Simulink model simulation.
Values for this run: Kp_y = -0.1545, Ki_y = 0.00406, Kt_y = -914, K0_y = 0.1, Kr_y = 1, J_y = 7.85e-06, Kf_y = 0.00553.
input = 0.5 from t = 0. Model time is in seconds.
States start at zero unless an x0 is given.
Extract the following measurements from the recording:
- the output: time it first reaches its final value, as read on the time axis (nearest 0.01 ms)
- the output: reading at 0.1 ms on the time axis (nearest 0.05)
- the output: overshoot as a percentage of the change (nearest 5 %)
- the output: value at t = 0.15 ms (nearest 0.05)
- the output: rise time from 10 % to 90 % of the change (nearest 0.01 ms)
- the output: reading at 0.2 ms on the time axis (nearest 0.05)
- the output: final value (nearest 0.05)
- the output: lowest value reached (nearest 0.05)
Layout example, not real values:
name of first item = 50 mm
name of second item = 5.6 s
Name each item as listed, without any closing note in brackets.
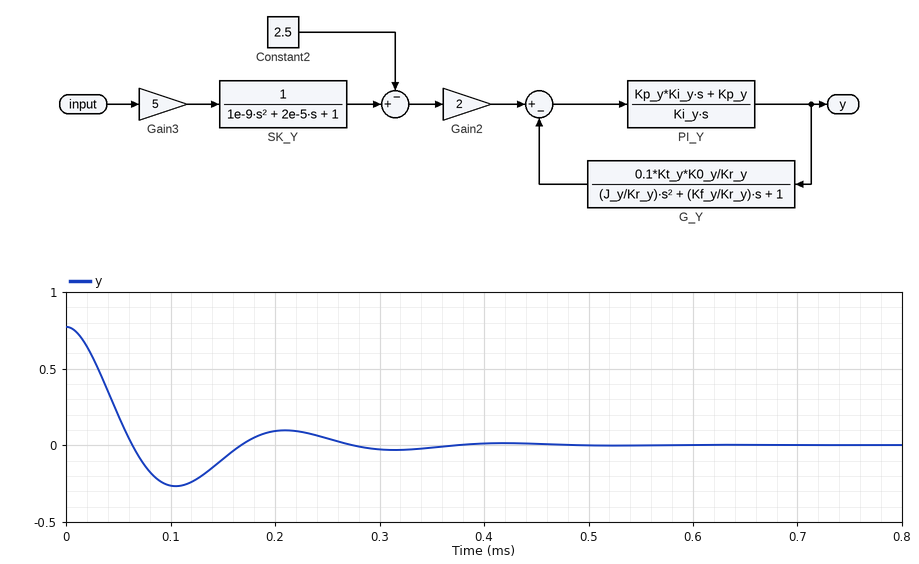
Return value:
the output: time it first reaches its final value, as read on the time axis = 0.06 ms
the output: reading at 0.1 ms on the time axis = -0.25
the output: overshoot as a percentage of the change = 35 %
the output: value at t = 0.15 ms = -0.10
the output: rise time from 10 % to 90 % of the change = 0.04 ms
the output: reading at 0.2 ms on the time axis = 0.10
the output: final value = 0.00
the output: lowest value reached = -0.25
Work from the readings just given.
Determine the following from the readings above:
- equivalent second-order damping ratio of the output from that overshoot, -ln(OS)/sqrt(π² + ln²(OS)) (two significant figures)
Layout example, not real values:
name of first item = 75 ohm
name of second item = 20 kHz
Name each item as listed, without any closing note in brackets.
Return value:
equivalent second-order damping ratio of the output from that overshoot, -ln(OS)/sqrt(π² + ln²(OS)) = 0.32
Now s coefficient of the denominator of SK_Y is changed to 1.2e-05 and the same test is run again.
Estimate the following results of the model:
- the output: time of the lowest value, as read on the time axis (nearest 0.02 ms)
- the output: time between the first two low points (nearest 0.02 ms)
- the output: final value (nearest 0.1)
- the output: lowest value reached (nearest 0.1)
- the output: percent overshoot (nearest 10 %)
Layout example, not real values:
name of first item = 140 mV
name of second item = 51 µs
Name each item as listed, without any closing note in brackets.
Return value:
the output: time of the lowest value, as read on the time axis = 0.10 ms
the output: time between the first two low points = 0.20 ms
the output: final value = 0.0
the output: lowest value reached = -0.4
the output: percent overshoot = 50 %
